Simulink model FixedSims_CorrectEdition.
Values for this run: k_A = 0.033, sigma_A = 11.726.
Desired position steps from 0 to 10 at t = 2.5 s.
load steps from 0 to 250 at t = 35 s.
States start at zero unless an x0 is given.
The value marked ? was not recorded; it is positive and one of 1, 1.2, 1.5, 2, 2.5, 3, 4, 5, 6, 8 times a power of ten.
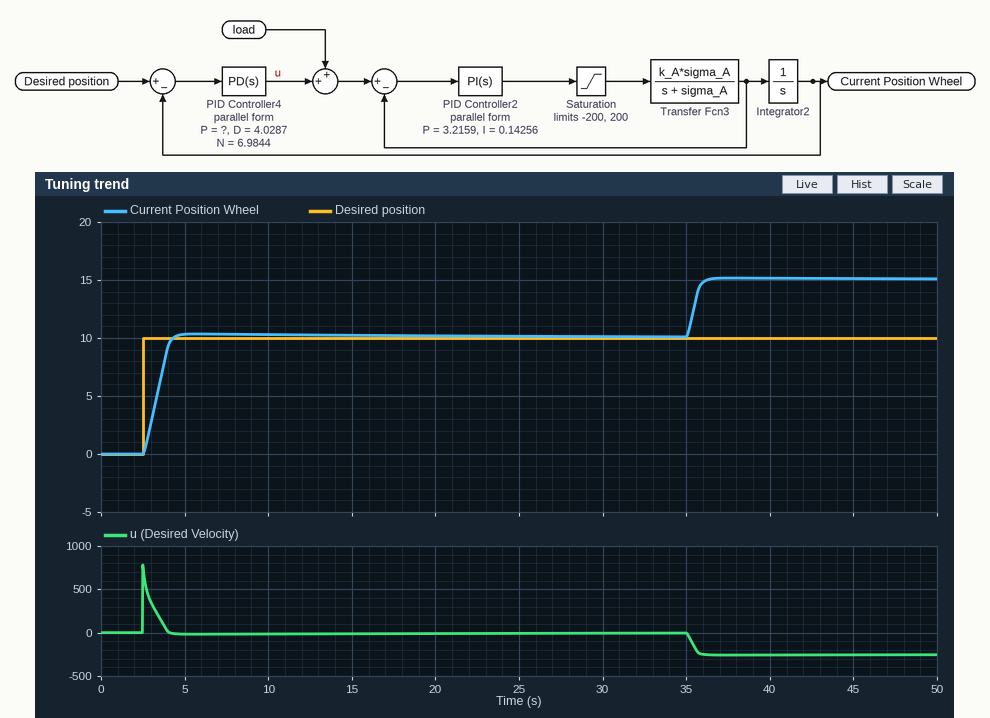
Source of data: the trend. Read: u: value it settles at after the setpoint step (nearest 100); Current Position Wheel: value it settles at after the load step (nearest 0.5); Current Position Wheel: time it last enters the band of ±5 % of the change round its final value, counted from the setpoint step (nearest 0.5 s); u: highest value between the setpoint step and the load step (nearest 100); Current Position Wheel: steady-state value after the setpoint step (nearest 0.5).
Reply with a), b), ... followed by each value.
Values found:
a) 0
b) 15.0
c) 1.5 s
d) 800
e) 10.0
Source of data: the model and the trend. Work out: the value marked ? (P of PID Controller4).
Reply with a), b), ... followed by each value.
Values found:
a) 50
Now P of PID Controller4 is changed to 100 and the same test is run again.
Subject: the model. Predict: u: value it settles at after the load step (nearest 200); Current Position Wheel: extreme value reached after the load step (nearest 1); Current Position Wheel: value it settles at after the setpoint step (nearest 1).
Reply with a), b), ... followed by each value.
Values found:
a) -200
b) 13
c) 10
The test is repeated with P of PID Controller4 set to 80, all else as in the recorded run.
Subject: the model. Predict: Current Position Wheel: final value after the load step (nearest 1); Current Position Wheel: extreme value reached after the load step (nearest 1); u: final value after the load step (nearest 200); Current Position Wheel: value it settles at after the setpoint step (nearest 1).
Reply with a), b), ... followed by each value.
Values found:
a) 13
b) 13
c) -200
d) 10
